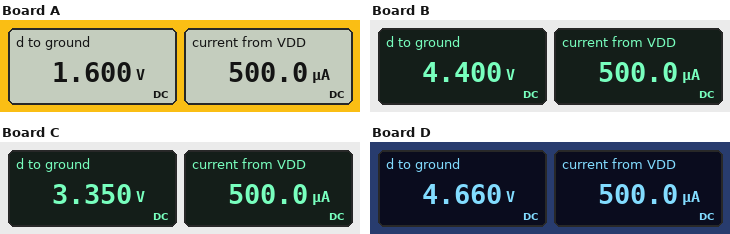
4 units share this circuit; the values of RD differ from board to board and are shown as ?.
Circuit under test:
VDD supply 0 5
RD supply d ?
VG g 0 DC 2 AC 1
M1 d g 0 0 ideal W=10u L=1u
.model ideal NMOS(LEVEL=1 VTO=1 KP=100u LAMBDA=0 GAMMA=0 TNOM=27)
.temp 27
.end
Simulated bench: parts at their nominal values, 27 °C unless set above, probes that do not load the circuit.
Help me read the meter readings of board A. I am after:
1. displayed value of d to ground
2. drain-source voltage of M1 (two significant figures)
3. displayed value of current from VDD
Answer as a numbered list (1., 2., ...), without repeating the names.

1. 1.600 V
2. 1.6 V
3. 500.0 µA
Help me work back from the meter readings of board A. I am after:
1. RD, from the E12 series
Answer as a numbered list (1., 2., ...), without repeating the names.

1. 6.8 kΩ
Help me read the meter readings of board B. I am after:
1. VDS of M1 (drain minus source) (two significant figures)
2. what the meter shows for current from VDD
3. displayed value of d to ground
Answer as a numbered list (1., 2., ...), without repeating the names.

1. 4.4 V
2. 500.0 µA
3. 4.400 V
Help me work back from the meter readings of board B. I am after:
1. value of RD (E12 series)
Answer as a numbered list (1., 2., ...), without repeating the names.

1. 1.2 kΩ
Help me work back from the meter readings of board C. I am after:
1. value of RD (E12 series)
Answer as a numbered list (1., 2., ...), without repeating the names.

1. 3.3 kΩ
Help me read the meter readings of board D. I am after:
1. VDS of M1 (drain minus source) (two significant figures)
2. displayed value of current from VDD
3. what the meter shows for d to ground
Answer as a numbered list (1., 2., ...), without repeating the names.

1. 4.7 V
2. 500.0 µA
3. 4.660 V
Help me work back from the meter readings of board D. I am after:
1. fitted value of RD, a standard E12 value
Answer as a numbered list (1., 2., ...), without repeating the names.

1. 680 Ω
